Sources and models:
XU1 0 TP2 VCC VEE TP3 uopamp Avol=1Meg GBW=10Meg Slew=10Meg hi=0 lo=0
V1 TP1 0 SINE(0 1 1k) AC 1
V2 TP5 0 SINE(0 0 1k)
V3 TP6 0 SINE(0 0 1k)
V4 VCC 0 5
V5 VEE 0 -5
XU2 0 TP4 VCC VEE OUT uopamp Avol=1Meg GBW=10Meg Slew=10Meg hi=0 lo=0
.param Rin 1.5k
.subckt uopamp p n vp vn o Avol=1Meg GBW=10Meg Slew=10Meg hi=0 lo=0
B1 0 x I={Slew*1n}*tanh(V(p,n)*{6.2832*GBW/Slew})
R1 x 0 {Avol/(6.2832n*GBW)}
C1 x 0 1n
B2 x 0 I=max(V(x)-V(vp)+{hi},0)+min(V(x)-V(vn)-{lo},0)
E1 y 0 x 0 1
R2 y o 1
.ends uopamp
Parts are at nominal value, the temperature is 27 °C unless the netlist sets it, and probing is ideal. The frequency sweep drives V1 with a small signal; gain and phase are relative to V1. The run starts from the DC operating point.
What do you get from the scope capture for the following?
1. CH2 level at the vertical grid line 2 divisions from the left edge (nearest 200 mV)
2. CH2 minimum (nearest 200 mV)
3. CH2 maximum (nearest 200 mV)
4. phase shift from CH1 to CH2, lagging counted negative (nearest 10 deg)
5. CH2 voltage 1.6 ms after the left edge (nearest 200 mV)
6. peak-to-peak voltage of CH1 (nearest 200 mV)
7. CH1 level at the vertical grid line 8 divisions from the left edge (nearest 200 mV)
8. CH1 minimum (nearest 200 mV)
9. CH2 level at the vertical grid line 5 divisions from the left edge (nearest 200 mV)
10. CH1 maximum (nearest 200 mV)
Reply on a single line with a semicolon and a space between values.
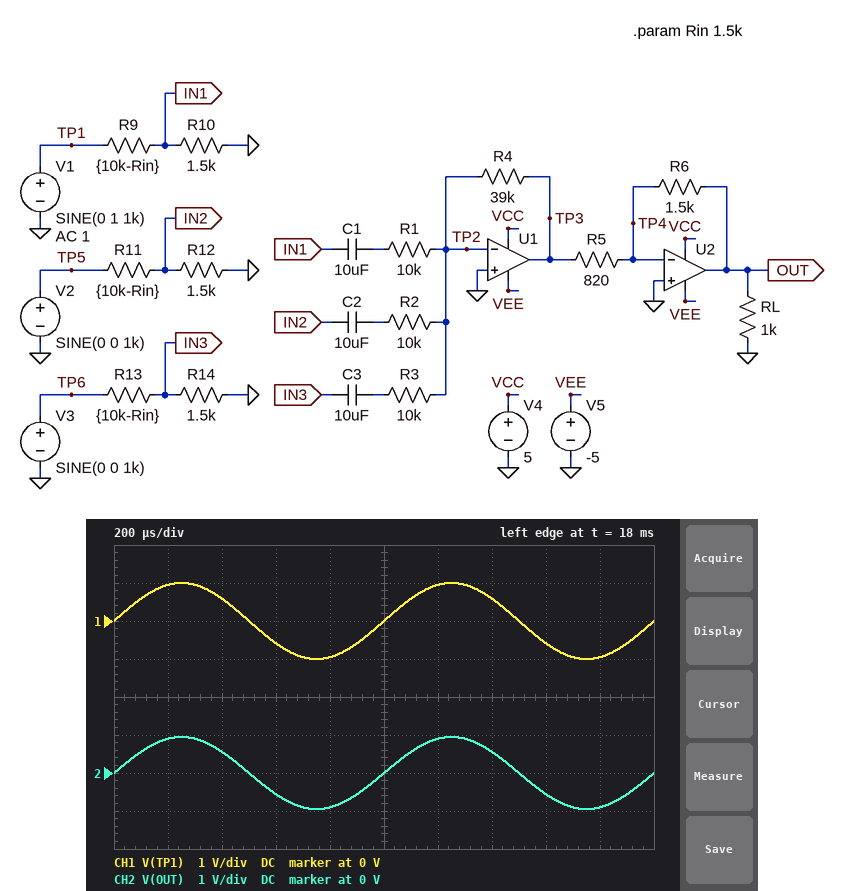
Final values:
600 mV; -1.0 V; 1.0 V; 0 deg; -600 mV; 2.0 V; -600 mV; -1.0 V; 0 V; 1.0 V
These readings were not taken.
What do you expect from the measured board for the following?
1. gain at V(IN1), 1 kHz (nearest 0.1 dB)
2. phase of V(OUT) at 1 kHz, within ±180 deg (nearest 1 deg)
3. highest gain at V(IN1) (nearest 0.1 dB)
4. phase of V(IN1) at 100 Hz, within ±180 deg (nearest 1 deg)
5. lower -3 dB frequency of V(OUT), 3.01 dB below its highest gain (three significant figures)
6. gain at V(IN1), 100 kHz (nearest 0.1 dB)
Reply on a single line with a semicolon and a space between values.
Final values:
-17.5 dB; 0 deg; -16.5 dB; 0 deg; 1.41 Hz; -17.5 dB
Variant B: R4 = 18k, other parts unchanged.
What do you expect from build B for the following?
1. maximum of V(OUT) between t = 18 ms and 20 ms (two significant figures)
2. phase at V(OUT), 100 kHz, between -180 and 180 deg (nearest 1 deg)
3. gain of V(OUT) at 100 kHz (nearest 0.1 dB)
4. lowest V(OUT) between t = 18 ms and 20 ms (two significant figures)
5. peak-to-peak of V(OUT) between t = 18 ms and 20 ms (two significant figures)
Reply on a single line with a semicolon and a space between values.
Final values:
440 mV; -5 deg; -7.2 dB; -440 mV; 880 mV
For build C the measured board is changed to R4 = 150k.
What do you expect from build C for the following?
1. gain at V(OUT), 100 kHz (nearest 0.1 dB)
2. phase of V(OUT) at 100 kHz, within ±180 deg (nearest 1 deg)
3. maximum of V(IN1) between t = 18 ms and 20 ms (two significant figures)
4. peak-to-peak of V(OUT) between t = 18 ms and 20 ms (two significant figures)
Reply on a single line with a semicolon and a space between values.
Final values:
10.6 dB; -24 deg; 130 mV; 7.3 V
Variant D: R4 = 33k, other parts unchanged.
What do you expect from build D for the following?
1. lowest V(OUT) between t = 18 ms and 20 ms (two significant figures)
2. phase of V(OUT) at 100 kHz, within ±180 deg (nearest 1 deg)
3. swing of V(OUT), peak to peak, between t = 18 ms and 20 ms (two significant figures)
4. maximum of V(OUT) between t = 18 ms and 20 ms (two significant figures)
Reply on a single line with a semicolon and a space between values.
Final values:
-800 mV; -7 deg; 1.6 V; 800 mV
